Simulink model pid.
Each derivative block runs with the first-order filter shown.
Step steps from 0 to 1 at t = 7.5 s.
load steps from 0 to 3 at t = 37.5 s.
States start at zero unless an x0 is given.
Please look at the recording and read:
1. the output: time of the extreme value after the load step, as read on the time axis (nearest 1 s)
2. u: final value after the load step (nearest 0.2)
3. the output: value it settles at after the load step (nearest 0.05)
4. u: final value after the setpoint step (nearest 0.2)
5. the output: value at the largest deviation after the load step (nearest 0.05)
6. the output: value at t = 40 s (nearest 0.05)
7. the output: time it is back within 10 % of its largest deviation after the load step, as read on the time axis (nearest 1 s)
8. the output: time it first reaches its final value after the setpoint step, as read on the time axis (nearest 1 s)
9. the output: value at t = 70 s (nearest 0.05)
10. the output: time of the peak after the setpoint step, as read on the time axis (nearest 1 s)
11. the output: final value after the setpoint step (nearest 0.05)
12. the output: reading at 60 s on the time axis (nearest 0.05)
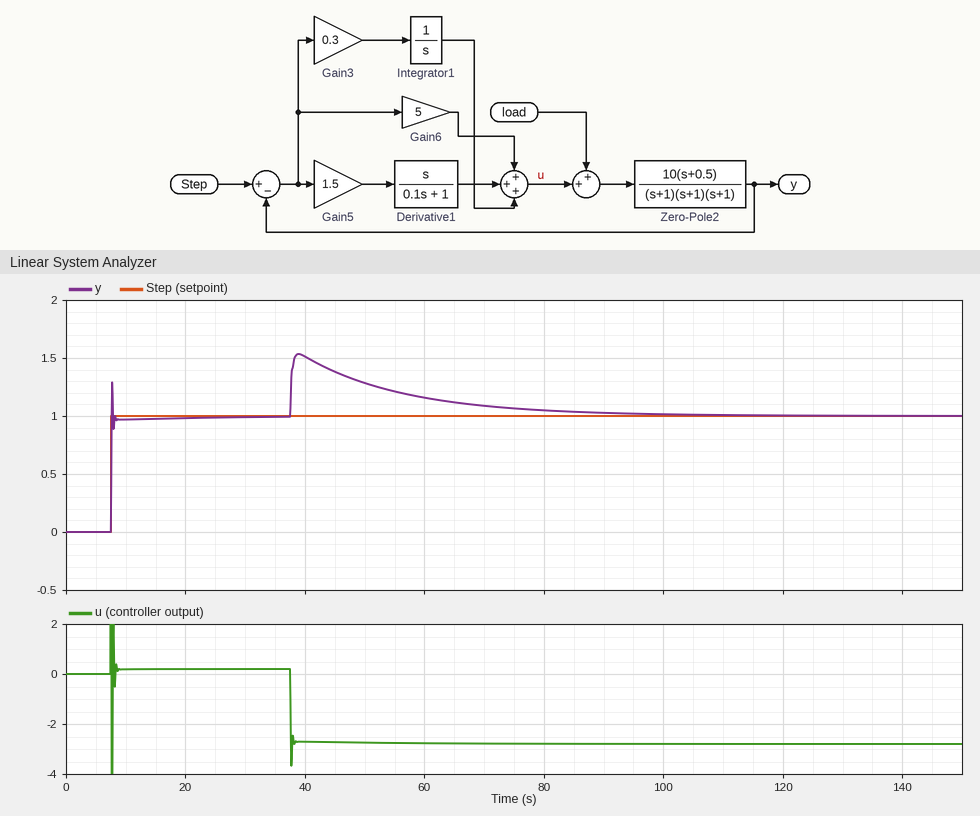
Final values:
39 s
-2.8
1.00
0.2
1.55
1.50
78 s
8 s
1.10
8 s
1.00
1.15
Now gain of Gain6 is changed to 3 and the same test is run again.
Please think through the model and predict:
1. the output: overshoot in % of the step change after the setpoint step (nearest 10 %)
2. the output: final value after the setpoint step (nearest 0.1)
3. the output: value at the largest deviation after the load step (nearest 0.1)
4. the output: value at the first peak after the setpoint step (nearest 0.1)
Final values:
20 %
1.0
1.8
1.2
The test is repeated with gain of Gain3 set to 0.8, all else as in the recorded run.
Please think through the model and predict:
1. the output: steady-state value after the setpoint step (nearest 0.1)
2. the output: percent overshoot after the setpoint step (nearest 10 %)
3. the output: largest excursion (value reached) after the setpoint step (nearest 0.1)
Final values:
1.0
30 %
1.3
